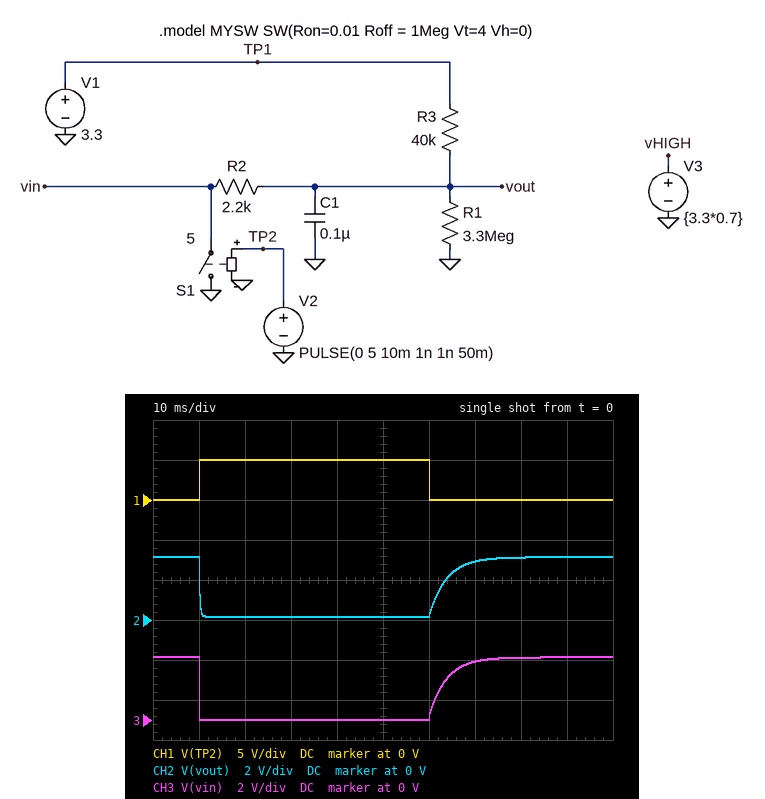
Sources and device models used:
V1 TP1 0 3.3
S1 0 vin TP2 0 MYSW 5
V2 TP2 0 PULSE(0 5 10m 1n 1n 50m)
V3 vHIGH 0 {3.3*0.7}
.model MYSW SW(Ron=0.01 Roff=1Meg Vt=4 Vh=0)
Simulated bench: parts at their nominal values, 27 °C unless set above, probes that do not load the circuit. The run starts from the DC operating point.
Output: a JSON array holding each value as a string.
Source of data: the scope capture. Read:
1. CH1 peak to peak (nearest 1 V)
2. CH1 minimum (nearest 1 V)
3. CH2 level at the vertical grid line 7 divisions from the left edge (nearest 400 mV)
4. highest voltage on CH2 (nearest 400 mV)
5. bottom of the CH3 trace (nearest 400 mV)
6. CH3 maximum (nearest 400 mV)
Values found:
["5 V", "0 V", "2.8 V", "3.2 V", "0 V", "3.2 V"]
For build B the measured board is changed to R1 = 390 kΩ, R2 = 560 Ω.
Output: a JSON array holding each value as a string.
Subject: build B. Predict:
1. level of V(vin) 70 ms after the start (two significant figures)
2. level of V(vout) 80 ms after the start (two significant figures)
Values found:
["2.7 V", "2.9 V"]
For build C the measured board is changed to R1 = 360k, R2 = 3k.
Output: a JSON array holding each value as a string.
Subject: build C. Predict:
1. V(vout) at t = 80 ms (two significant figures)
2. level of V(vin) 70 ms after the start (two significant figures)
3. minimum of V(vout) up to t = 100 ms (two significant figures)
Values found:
["2.9 V", "2.7 V", "230 mV"]
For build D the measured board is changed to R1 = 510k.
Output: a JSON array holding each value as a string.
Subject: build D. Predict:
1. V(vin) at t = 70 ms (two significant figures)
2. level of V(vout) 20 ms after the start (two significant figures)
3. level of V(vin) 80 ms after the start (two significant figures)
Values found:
["2.8 V", "170 mV", "2.9 V"]
